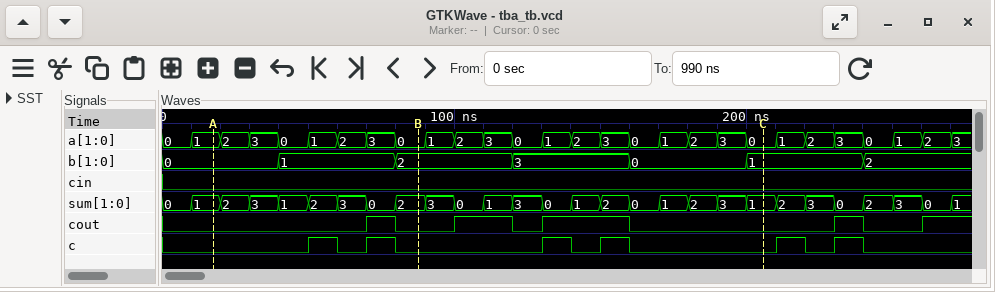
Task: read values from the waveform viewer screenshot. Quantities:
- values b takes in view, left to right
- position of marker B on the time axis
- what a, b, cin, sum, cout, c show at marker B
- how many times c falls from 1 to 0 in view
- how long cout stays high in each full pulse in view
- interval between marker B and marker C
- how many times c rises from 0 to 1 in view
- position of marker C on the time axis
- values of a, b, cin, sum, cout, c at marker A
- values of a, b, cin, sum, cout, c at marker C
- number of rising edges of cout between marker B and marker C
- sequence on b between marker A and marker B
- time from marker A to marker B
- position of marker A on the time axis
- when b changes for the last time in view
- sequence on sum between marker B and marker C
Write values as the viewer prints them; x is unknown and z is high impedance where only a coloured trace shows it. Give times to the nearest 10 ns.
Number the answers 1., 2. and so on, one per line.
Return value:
1. 0, 1, 2, 3, 0, 1, 2
2. 90 ns
3. a=0, b=2, cin=0, sum=2, cout=0, c=0
4. 6
5. 10 ns, 20 ns, 30 ns, 10 ns
6. 120 ns
7. 6
8. 210 ns
9. a=1, b=0, cin=0, sum=1, cout=0, c=0
10. a=0, b=1, cin=0, sum=1, cout=0, c=0
11. 2
12. 0, 1, 2
13. 70 ns
14. 20 ns
15. 240 ns
16. 2, 3, 0, 1, 3, 0, 1, 2, 0, 1, 2, 3, 1
